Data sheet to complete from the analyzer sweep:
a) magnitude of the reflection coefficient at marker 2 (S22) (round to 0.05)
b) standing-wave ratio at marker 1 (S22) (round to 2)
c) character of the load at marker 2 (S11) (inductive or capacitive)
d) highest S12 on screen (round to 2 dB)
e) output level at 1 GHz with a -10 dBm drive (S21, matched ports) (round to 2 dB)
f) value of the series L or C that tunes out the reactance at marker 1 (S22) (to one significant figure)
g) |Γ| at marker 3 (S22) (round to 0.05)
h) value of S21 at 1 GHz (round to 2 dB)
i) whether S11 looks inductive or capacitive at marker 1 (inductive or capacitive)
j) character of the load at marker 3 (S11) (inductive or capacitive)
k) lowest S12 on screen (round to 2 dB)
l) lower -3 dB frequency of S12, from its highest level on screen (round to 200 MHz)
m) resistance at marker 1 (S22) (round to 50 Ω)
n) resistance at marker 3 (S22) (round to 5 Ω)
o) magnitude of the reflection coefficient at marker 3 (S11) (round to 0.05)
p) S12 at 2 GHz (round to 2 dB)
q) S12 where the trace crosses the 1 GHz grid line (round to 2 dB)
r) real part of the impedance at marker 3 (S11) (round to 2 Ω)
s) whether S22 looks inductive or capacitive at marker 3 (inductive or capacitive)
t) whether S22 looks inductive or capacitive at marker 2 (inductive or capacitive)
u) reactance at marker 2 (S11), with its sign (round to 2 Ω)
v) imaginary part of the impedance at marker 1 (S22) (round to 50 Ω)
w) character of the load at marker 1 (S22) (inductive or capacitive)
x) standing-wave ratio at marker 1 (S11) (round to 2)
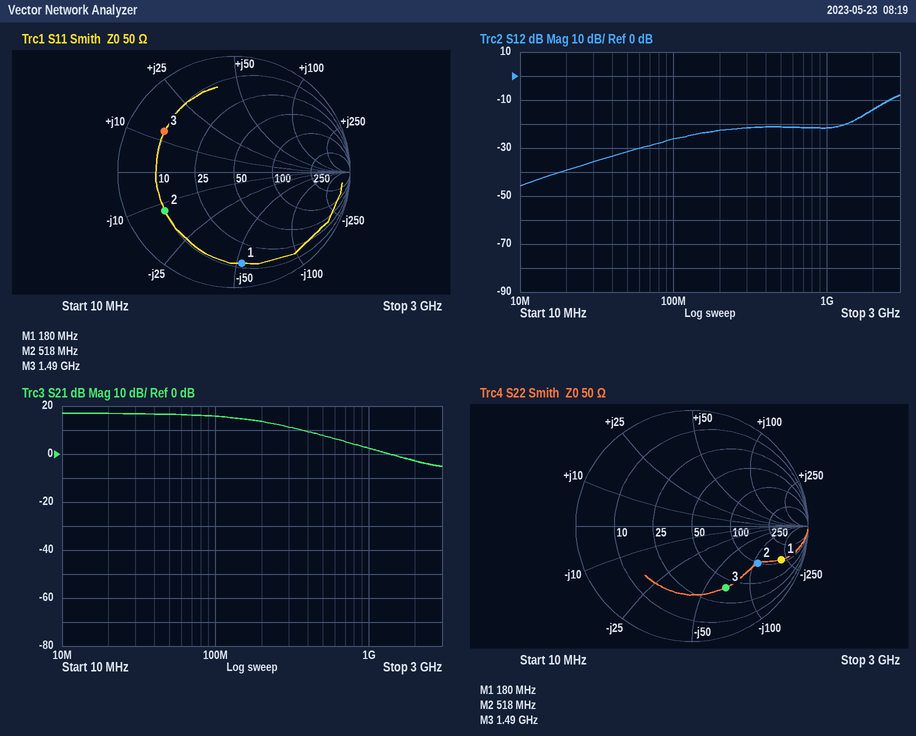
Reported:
0.65
10
capacitive
-8 dB
-8 dBm
200 nH
0.60
2 dB
capacitive
inductive
-46 dB
2.4 GHz
100 Ω
40 Ω
0.70
-14 dB
-22 dB
10 Ω
capacitive
capacitive
-12 Ω
-200 Ω
capacitive
8
